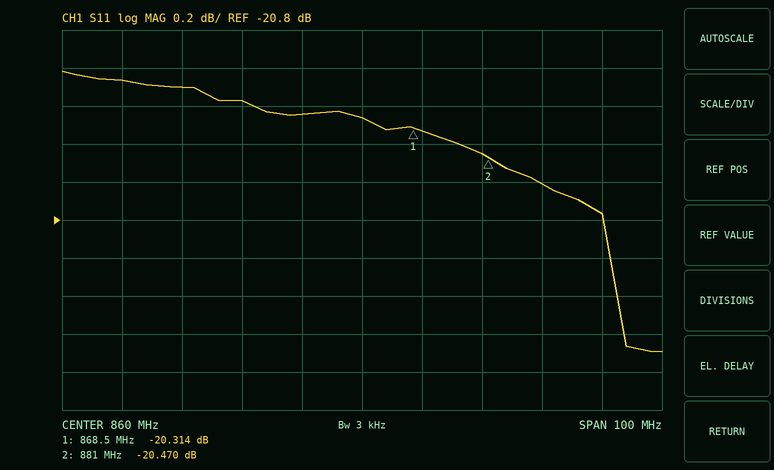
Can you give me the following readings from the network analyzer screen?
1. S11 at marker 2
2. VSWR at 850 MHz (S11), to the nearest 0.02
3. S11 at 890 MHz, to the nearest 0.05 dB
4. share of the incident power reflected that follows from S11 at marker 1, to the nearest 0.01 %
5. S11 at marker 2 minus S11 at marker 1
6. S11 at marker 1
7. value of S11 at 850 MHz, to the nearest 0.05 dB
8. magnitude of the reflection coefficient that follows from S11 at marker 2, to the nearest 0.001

-20.470 dB
1.22
-20.60 dB
0.93 %
-0.156 dB
-20.314 dB
-20.25 dB
0.095
